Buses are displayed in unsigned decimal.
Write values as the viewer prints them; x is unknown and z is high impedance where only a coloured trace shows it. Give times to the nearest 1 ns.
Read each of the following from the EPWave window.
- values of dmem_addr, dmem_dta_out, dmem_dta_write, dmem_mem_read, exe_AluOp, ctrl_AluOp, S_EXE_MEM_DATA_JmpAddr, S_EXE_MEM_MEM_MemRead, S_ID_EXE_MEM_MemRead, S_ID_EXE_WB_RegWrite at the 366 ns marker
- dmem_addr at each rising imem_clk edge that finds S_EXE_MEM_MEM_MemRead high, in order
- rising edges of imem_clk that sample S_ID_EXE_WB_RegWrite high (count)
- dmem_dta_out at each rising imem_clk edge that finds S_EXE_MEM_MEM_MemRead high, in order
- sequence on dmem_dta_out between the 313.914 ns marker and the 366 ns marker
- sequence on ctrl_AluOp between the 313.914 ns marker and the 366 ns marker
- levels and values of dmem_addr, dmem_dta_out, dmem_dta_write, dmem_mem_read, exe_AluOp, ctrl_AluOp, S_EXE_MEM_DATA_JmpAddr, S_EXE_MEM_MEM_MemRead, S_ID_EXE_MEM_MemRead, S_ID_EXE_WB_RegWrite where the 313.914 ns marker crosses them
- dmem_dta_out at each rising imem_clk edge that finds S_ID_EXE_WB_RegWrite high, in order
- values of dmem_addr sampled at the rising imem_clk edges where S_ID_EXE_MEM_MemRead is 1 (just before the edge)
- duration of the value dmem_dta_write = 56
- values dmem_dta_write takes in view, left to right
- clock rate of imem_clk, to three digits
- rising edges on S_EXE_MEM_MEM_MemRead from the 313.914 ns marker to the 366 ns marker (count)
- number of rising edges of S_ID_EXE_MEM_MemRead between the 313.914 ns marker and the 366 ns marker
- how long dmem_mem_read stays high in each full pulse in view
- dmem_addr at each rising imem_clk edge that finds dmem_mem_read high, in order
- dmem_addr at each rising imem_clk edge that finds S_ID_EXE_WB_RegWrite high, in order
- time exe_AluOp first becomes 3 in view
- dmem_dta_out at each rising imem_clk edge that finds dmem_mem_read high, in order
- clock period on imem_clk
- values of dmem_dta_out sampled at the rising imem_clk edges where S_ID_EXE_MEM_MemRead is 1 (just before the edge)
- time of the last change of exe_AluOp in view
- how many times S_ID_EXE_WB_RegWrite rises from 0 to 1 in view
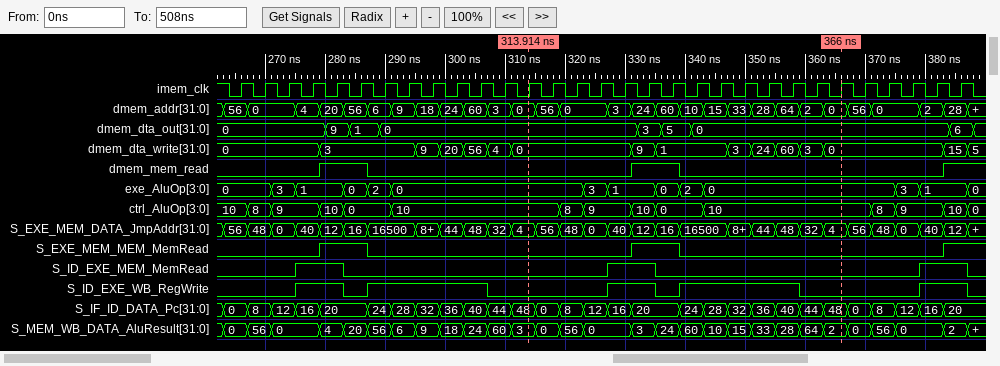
dmem_addr=0, dmem_dta_out=0, dmem_dta_write=0, dmem_mem_read=0, exe_AluOp=0, ctrl_AluOp=10, S_EXE_MEM_DATA_JmpAddr=4, S_EXE_MEM_MEM_MemRead=0, S_ID_EXE_MEM_MemRead=0, S_ID_EXE_WB_RegWrite=0
20, 56, 24, 60, 28
16
9, 1, 3, 5, 6
0, 3, 5, 0
10, 8, 9, 10, 0, 10
dmem_addr=0, dmem_dta_out=0, dmem_dta_write=0, dmem_mem_read=0, exe_AluOp=0, ctrl_AluOp=10, S_EXE_MEM_DATA_JmpAddr=4, S_EXE_MEM_MEM_MemRead=0, S_ID_EXE_MEM_MemRead=0, S_ID_EXE_WB_RegWrite=0
0, 9, 0, 0, 0, 0, 0, 0, 3, 0, 0, 0, 0, 0, 0, 6
4, 20, 3, 24, 2, 28
4 ns
0, 3, 9, 20, 56, 4, 0, 9, 1, 3, 24, 60, 3, 0, 15, 5
250 MHz
1
1
8 ns, 8 ns
20, 56, 24, 60, 28
4, 20, 6, 9, 18, 24, 60, 3, 24, 10, 15, 33, 28, 64, 2, 28
271 ns
9, 1, 3, 5, 6
4 ns
0, 9, 0, 3, 0, 6
387 ns
5
